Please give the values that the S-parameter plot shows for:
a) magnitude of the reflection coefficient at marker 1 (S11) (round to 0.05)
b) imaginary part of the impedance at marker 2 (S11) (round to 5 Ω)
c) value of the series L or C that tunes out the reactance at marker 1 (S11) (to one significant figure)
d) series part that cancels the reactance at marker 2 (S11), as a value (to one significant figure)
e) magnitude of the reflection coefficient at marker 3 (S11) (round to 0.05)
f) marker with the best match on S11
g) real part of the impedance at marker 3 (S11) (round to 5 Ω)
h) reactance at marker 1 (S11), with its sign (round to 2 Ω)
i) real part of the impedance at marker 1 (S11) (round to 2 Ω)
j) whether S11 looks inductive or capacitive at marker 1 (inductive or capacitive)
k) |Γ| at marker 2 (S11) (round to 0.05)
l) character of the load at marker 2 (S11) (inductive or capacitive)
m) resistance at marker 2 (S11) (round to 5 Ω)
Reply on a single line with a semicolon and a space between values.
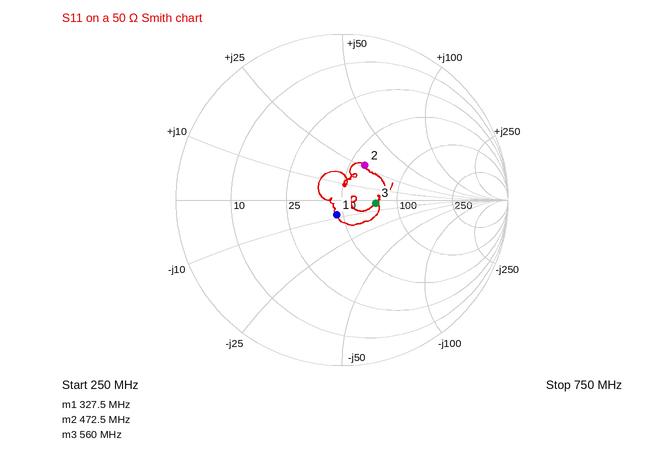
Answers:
0.10; +25 Ω; 4 nH; 10 pF; 0.20; marker 1; 75 Ω; -8 Ω; 46 Ω; capacitive; 0.25; inductive; 60 Ω
